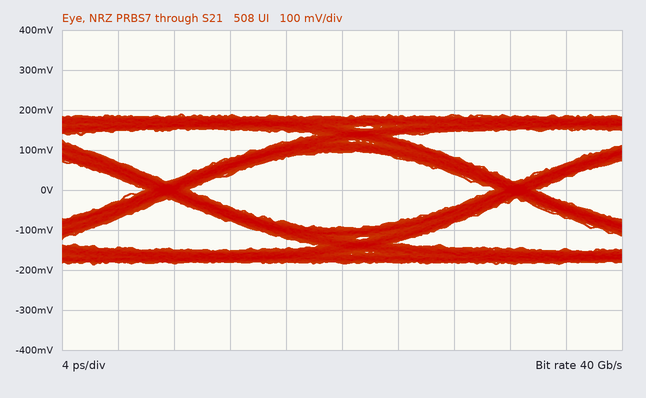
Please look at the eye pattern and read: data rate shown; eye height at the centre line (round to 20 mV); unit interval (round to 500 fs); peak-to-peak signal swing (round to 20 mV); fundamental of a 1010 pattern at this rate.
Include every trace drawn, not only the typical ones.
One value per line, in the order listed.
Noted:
40 Gb/s
180 mV
25.0 ps
380 mV
20 GHz
